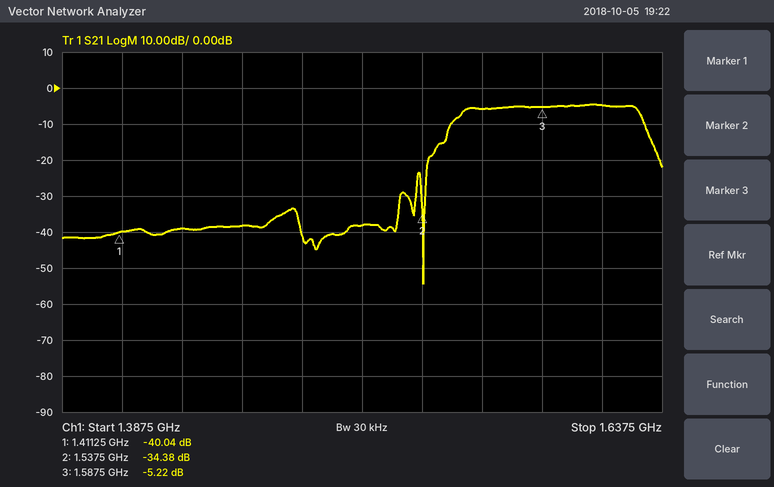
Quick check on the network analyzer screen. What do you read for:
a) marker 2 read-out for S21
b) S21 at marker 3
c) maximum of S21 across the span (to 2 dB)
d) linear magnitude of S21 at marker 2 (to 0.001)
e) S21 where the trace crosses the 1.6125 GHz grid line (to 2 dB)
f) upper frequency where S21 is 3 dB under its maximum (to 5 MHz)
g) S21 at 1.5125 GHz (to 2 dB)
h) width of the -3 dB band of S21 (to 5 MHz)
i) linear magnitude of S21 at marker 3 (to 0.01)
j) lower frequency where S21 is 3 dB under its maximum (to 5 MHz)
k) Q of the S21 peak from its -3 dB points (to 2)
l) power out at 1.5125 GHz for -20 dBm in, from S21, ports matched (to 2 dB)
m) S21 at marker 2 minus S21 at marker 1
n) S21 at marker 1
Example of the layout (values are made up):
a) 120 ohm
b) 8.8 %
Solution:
a) -34.38 dB
b) -5.22 dB
c) -4 dB
d) 0.019
e) -4 dB
f) 1.630 GHz
g) -38 dB
h) 75 MHz
i) 0.55
j) 1.555 GHz
k) 22
l) -58 dBm
m) 5.66 dB
n) -40.04 dB
